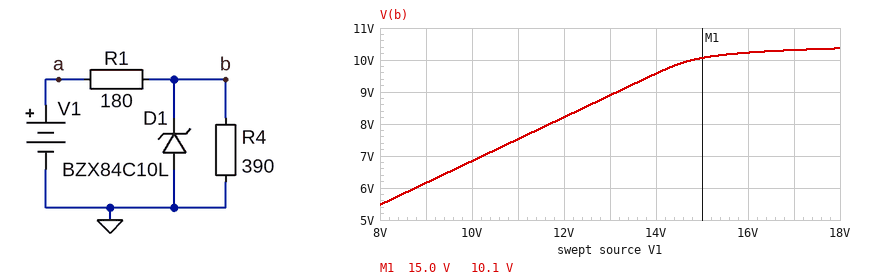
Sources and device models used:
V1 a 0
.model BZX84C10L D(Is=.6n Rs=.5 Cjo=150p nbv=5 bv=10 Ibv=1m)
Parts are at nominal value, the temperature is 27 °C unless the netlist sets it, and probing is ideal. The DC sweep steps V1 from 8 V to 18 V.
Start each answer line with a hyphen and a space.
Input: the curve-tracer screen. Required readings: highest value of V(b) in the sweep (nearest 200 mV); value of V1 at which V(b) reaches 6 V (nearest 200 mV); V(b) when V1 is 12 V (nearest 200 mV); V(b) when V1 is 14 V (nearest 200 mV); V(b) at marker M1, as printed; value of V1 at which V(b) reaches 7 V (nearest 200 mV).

- 10.4 V
- 8.8 V
- 8.2 V
- 9.6 V
- 10.1 V
- 10.2 V
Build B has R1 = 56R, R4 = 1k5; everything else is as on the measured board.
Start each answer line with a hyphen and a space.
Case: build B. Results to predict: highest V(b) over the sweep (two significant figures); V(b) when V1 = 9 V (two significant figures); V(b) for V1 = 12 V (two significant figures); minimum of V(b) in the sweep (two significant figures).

- 11 V
- 8.7 V
- 10 V
- 7.7 V
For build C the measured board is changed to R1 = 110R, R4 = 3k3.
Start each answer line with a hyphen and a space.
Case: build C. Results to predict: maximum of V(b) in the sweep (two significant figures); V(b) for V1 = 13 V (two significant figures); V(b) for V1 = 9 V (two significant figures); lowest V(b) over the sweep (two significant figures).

- 11 V
- 10 V
- 8.7 V
- 7.7 V
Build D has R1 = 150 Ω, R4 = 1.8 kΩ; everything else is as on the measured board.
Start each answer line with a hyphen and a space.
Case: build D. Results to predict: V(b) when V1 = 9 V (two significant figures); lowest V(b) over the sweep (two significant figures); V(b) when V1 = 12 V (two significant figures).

- 8.3 V
- 7.4 V
- 10 V
